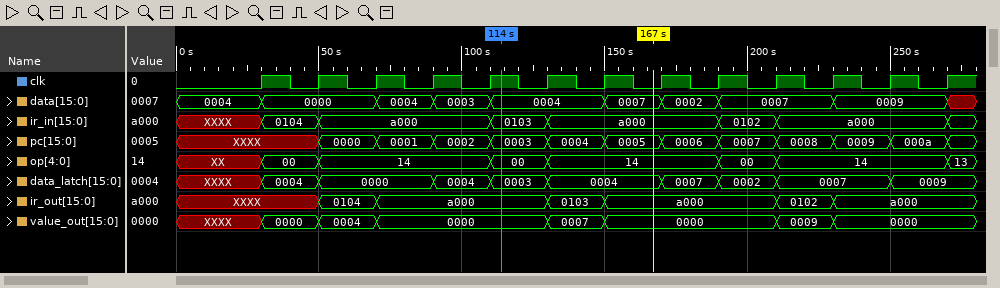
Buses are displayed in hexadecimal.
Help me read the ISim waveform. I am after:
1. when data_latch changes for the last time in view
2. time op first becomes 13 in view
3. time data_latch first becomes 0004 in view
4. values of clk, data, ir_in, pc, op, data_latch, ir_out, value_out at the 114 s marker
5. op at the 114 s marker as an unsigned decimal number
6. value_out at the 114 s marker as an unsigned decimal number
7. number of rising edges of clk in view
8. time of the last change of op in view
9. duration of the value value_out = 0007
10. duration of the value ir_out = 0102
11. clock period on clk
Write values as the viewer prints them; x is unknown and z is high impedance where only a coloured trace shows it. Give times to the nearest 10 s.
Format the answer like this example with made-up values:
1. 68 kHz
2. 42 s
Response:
1. 250 s
2. 270 s
3. 30 s
4. clk=1, data=0004, ir_in=0103, pc=0003, op=00, data_latch=0003, ir_out=a000, value_out=0000
5. 0
6. 0
7. 13
8. 270 s
9. 20 s
10. 20 s
11. 20 s
